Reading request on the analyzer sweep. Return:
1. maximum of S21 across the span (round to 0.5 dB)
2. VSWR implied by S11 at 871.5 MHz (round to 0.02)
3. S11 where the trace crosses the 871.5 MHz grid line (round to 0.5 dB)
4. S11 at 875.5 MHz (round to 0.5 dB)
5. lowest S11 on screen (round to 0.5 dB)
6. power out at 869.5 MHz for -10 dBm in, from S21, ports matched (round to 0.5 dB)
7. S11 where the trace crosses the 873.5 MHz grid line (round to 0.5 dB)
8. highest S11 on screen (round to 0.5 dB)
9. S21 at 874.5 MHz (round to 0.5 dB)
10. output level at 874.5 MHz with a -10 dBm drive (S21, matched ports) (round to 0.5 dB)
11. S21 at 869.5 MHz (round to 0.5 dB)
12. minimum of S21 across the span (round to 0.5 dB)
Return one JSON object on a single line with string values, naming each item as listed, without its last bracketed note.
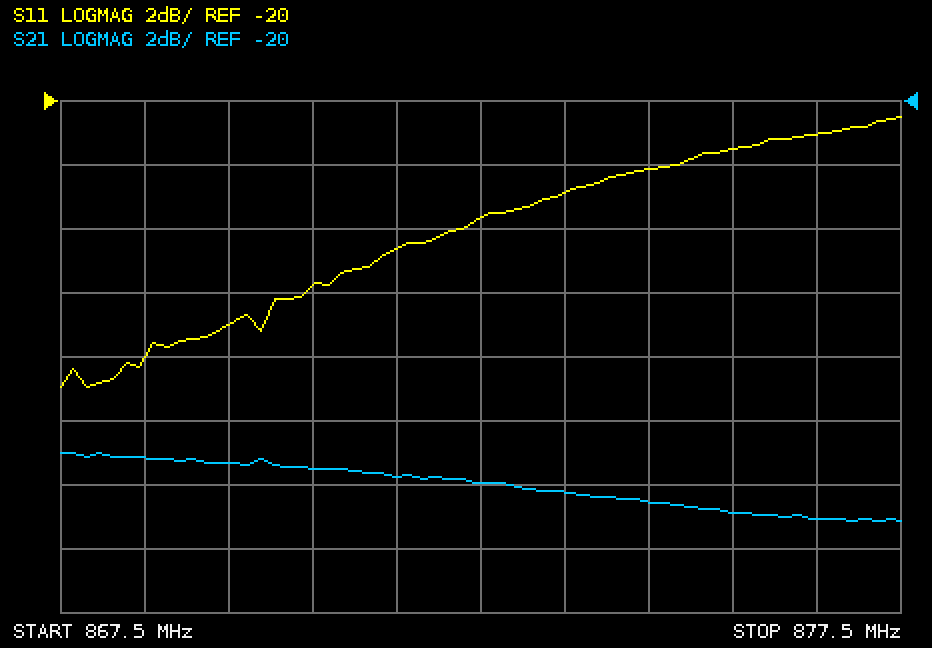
{"maximum of S21 across the span": "-31.0 dB", "VSWR implied by S11 at 871.5 MHz": "1.12", "S11 where the trace crosses the 871.5 MHz grid line": "-24.5 dB", "S11 at 875.5 MHz": "-21.5 dB", "lowest S11 on screen": "-29.0 dB", "power out at 869.5 MHz for -10 dBm in, from S21, ports matched": "-41.5 dBm", "S11 where the trace crosses the 873.5 MHz grid line": "-23.0 dB", "highest S11 on screen": "-20.5 dB", "S21 at 874.5 MHz": "-32.5 dB", "output level at 874.5 MHz with a -10 dBm drive (S21, matched ports)": "-42.5 dBm", "S21 at 869.5 MHz": "-31.5 dB", "minimum of S21 across the span": "-33.0 dB"}
